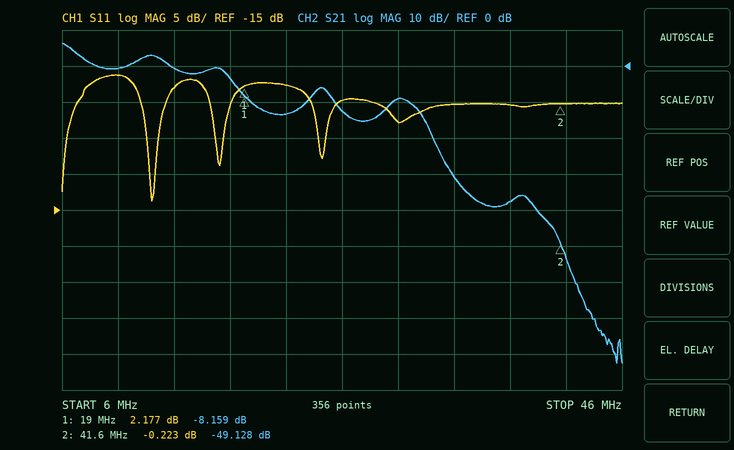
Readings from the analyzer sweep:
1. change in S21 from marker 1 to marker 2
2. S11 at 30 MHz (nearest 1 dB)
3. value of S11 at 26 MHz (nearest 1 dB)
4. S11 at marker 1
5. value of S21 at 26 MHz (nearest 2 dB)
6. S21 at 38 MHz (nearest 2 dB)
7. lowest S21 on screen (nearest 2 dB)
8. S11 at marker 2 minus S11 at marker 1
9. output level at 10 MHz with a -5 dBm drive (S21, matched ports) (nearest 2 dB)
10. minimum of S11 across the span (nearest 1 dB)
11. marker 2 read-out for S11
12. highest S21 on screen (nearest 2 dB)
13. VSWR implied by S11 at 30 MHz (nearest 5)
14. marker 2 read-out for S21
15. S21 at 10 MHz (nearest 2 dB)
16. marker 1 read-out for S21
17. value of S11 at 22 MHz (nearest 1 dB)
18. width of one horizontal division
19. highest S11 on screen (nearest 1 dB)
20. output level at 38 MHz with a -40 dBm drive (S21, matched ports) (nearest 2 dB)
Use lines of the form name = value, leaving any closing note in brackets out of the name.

change in S21 from marker 1 to marker 2 = -40.969 dB
S11 at 30 MHz = -3 dB
value of S11 at 26 MHz = 0 dB
S11 at marker 1 = 2.177 dB
value of S21 at 26 MHz = -12 dB
S21 at 38 MHz = -38 dB
lowest S21 on screen = -82 dB
S11 at marker 2 minus S11 at marker 1 = -2.400 dB
output level at 10 MHz with a -5 dBm drive (S21, matched ports) = -6 dBm
minimum of S11 across the span = -14 dB
marker 2 read-out for S11 = -0.223 dB
highest S21 on screen = 6 dB
VSWR implied by S11 at 30 MHz = 5
marker 2 read-out for S21 = -49.128 dB
S21 at 10 MHz = 0 dB
marker 1 read-out for S21 = -8.159 dB
value of S11 at 22 MHz = 2 dB
width of one horizontal division = 4 MHz
highest S11 on screen = 4 dB
output level at 38 MHz with a -40 dBm drive (S21, matched ports) = -78 dBm
